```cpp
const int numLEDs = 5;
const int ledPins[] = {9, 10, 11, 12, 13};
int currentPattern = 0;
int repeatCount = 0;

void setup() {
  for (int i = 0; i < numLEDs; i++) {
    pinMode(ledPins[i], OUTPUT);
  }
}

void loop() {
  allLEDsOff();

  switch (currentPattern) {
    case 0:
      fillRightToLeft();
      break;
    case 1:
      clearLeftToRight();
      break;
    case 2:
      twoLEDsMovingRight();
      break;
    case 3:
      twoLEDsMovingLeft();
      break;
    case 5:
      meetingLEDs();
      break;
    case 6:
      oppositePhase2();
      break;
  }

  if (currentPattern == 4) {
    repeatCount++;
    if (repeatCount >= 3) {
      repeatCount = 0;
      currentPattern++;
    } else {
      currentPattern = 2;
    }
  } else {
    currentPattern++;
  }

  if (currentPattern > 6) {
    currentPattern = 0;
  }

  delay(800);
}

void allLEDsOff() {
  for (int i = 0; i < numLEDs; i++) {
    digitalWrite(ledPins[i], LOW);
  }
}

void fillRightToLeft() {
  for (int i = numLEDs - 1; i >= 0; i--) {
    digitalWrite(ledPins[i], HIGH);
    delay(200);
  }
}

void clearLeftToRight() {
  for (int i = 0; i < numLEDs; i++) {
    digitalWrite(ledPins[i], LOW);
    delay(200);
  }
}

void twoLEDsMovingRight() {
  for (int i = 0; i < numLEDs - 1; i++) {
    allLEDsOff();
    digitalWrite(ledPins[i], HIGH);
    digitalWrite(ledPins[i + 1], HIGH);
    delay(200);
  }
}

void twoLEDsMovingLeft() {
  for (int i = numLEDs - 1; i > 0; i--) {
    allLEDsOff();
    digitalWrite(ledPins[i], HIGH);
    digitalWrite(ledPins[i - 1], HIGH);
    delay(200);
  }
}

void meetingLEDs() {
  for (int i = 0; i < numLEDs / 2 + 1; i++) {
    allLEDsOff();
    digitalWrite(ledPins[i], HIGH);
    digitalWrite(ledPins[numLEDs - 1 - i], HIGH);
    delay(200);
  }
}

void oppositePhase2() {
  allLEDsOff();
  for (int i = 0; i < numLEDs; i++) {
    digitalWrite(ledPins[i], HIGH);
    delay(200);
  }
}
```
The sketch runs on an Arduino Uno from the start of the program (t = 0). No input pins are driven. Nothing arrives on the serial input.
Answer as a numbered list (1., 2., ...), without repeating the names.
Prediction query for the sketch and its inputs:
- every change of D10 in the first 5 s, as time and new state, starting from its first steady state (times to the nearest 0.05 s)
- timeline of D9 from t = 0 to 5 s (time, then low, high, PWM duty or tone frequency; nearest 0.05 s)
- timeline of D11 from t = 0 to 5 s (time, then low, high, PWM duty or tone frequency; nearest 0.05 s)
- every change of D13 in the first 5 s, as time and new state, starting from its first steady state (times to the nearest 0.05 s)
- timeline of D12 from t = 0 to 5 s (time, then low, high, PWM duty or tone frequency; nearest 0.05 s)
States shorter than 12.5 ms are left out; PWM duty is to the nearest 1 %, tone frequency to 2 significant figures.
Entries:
1. 0 s low; 0.6 s high; 1.8 s low; 3.6 s high; 4 s low
2. 0 s low; 0.8 s high; 1.8 s low; 3.6 s high; 3.8 s low
3. 0 s low; 0.4 s high; 1.8 s low; 3.8 s high; 4.2 s low
4. 0 s high; 1.8 s low; 4.2 s high
5. 0 s low; 0.2 s high; 1.8 s low; 4 s high
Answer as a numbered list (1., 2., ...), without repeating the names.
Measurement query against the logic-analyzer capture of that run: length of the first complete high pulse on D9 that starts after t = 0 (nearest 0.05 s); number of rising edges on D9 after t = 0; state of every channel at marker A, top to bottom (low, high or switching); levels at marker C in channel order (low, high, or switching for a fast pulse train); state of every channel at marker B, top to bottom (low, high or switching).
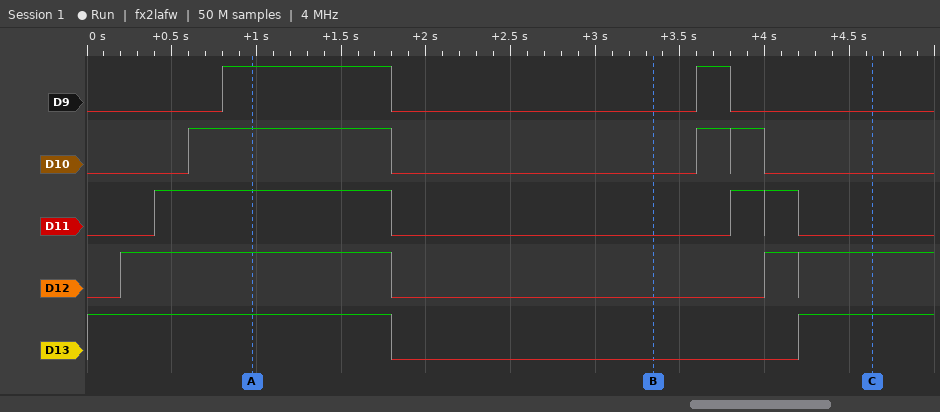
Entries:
1. 1.00 s
2. 2
3. D9 high, D10 high, D11 high, D12 high, D13 high
4. D9 low, D10 low, D11 low, D12 high, D13 high
5. D9 low, D10 low, D11 low, D12 low, D13 low
